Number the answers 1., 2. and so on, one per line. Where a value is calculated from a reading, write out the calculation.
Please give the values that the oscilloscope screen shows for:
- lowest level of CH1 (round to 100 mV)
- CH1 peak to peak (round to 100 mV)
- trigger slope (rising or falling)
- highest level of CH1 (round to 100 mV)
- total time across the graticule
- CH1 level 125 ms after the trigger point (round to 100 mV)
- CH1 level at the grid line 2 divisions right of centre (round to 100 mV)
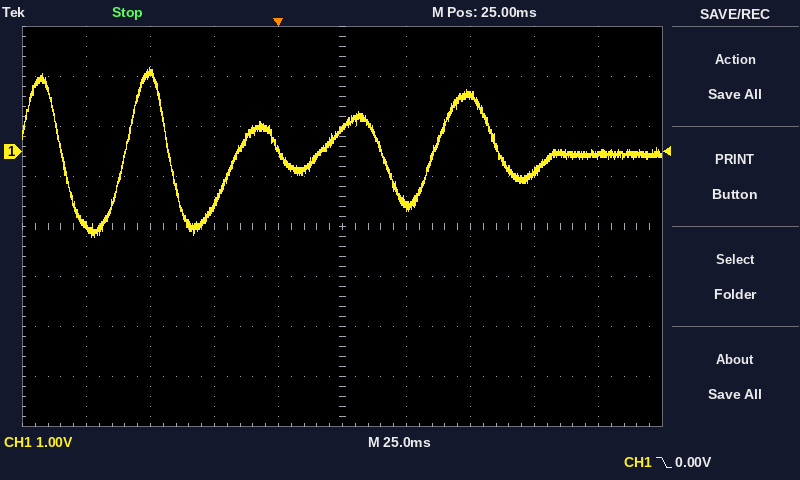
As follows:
1. -1.7 V
2. 1.7 V − (-1.7 V) = 3.4 V
3. falling
4. 1.7 V
5. 250 ms
6. -100 mV
7. 1.1 V
